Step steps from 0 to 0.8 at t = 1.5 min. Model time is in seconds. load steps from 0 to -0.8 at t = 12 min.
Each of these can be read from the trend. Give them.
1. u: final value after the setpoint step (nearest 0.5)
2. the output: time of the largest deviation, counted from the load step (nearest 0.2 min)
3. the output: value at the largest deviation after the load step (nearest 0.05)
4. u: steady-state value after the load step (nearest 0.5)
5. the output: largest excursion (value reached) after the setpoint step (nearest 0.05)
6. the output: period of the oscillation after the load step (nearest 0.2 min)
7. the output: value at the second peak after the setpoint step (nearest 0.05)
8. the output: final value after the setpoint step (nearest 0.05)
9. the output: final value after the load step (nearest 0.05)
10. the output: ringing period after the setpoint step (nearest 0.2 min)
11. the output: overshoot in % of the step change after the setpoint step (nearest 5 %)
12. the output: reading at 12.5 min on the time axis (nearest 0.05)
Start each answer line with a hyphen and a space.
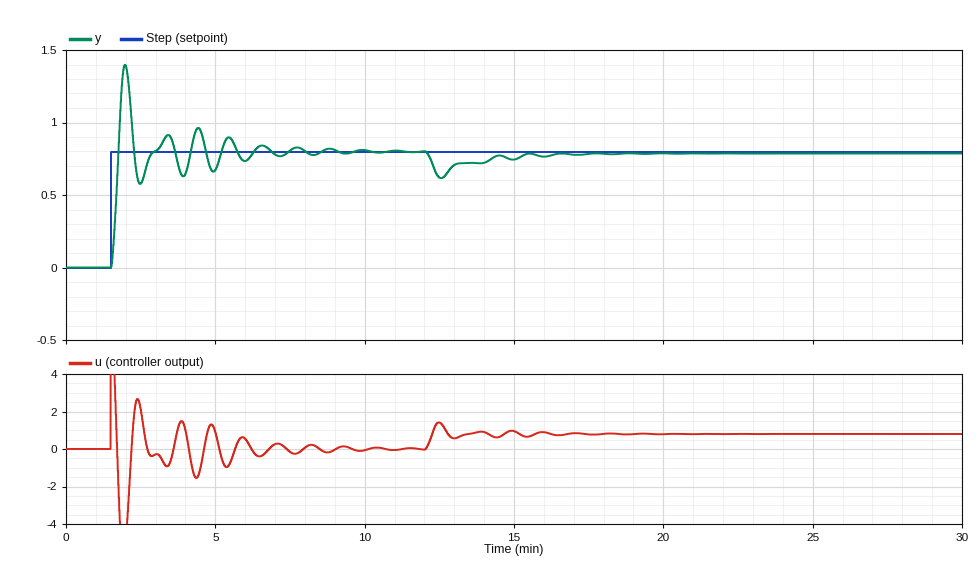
- 0.0
- 0.6 min
- 0.60
- 1.0
- 1.40
- 2.4 min
- 0.90
- 0.80
- 0.80
- 1.4 min
- 75 %
- 0.60
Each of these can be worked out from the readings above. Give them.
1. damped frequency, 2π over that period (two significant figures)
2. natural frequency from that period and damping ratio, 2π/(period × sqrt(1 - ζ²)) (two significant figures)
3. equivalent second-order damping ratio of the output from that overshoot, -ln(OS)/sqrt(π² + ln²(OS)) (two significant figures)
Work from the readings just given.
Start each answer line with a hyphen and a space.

- 4.5 rad/min
- 4.5 rad/min
- 0.091
